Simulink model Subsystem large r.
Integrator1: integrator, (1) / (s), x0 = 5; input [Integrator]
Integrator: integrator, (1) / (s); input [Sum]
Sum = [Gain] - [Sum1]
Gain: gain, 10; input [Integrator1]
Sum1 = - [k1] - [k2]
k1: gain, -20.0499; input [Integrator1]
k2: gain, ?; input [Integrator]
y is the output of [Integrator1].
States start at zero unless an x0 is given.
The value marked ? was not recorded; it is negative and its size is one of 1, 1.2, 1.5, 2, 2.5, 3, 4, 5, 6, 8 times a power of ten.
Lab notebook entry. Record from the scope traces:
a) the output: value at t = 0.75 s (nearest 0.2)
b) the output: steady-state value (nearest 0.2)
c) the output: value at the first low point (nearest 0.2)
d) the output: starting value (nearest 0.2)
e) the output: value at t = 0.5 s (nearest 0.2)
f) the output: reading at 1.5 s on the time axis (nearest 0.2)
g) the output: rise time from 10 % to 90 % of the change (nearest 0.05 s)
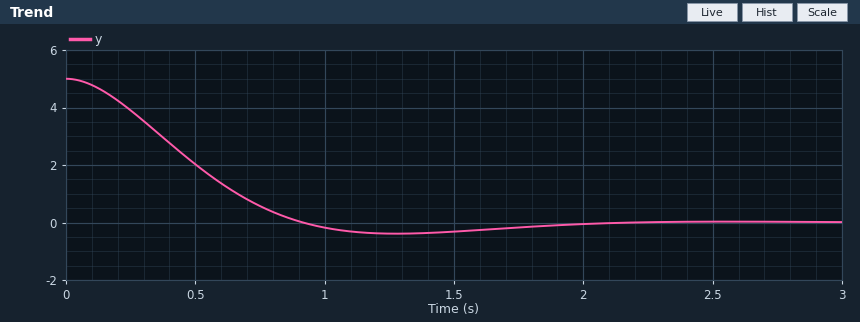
0.6
0.0
-0.4
5.0
2.0
-0.4
0.60 s
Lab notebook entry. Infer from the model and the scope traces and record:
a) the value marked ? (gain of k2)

-4
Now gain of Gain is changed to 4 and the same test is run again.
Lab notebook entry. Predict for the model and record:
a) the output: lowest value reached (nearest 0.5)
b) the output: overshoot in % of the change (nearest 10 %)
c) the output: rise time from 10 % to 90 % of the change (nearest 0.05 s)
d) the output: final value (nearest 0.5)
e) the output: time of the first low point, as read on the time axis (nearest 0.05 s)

-1.0
20 %
0.40 s
0.0
0.90 s
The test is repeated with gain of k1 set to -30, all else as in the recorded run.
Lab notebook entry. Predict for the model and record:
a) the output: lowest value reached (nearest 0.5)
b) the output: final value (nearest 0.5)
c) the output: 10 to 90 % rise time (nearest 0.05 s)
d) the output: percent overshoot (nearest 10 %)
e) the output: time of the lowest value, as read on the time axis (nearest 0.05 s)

-1.0
0.0
0.35 s
20 %
0.80 s
